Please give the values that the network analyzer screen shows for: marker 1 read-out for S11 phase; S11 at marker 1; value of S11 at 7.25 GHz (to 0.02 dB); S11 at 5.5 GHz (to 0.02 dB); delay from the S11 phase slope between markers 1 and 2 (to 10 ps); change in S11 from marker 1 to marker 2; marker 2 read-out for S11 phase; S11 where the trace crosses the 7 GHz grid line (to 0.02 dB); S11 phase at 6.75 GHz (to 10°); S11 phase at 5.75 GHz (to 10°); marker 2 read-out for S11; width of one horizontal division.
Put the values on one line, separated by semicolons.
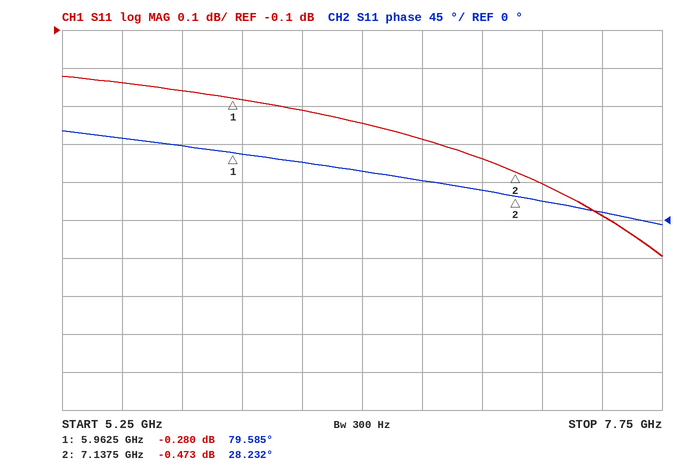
79.585°; -0.280 dB; -0.50 dB; -0.24 dB; 120 ps; -0.193 dB; 28.232°; -0.44 dB; 50°; 90°; -0.473 dB; 250 MHz
